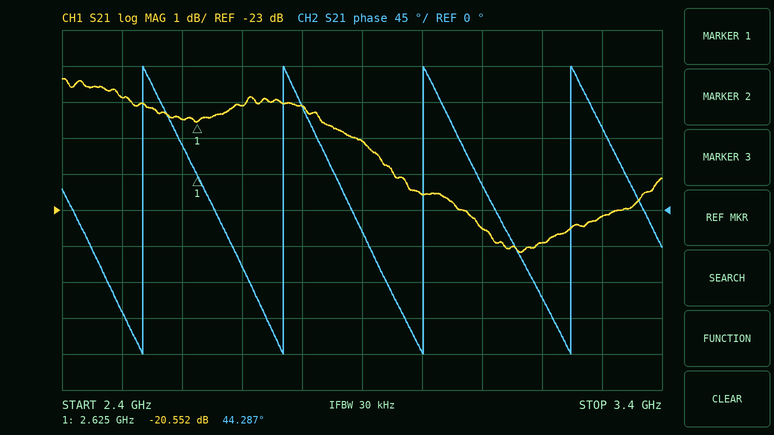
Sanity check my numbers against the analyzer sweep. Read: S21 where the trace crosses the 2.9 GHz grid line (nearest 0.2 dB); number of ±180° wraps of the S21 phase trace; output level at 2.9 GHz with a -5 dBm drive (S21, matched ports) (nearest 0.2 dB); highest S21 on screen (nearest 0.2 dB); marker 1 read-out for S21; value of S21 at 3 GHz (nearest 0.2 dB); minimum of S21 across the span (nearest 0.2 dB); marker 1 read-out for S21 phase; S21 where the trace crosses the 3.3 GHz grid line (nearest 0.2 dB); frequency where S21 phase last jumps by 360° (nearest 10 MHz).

-21.0 dB
4
-26.0 dBm
-19.4 dB
-20.552 dB
-22.6 dB
-24.2 dB
44.287°
-23.2 dB
3.25 GHz
